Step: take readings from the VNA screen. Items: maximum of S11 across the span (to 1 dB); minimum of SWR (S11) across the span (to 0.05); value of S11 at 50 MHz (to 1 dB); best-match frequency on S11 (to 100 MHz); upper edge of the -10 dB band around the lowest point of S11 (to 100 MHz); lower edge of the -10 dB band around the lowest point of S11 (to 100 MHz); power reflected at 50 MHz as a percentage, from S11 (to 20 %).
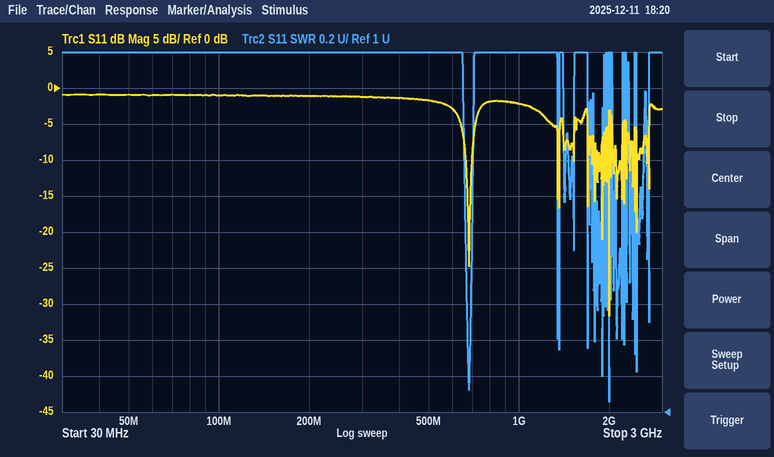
-1 dB
1.05
-1 dB
2.0 GHz
2.0 GHz
2.0 GHz
80 %
